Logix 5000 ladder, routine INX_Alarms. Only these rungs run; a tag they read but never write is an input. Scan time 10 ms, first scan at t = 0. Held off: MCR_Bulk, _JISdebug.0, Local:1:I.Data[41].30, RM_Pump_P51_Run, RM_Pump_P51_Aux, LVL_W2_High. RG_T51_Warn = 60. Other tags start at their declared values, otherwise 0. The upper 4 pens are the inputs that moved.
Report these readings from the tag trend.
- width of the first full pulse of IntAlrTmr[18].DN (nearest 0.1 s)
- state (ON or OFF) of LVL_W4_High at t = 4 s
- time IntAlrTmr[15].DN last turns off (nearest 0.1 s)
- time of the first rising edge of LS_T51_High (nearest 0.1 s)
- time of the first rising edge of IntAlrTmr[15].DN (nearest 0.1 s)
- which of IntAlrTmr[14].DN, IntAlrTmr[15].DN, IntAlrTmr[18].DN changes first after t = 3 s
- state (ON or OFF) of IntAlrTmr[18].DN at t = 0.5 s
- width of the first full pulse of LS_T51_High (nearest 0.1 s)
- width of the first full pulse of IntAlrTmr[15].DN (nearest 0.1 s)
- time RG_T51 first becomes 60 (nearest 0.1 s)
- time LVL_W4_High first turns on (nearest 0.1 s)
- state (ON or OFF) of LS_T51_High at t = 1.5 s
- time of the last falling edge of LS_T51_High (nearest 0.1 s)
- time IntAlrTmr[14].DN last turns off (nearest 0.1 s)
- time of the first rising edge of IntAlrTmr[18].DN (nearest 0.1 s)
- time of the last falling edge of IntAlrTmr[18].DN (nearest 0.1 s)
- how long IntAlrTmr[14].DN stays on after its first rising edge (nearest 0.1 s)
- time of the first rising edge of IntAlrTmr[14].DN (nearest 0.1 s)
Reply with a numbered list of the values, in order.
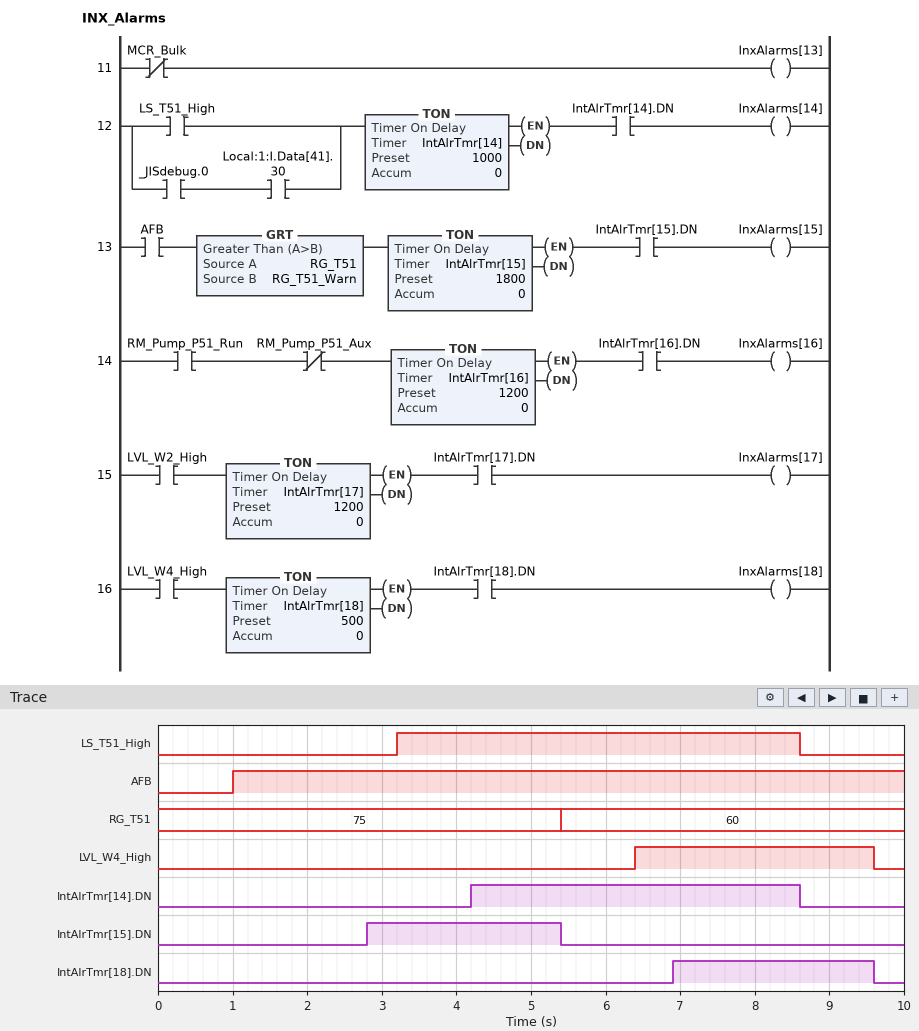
1. 2.7 s
2. OFF
3. 5.4 s
4. 3.2 s
5. 2.8 s
6. IntAlrTmr[14].DN
7. OFF
8. 5.4 s
9. 2.6 s
10. 5.4 s
11. 6.4 s
12. OFF
13. 8.6 s
14. 8.6 s
15. 6.9 s
16. 9.6 s
17. 4.4 s
18. 4.2 s
